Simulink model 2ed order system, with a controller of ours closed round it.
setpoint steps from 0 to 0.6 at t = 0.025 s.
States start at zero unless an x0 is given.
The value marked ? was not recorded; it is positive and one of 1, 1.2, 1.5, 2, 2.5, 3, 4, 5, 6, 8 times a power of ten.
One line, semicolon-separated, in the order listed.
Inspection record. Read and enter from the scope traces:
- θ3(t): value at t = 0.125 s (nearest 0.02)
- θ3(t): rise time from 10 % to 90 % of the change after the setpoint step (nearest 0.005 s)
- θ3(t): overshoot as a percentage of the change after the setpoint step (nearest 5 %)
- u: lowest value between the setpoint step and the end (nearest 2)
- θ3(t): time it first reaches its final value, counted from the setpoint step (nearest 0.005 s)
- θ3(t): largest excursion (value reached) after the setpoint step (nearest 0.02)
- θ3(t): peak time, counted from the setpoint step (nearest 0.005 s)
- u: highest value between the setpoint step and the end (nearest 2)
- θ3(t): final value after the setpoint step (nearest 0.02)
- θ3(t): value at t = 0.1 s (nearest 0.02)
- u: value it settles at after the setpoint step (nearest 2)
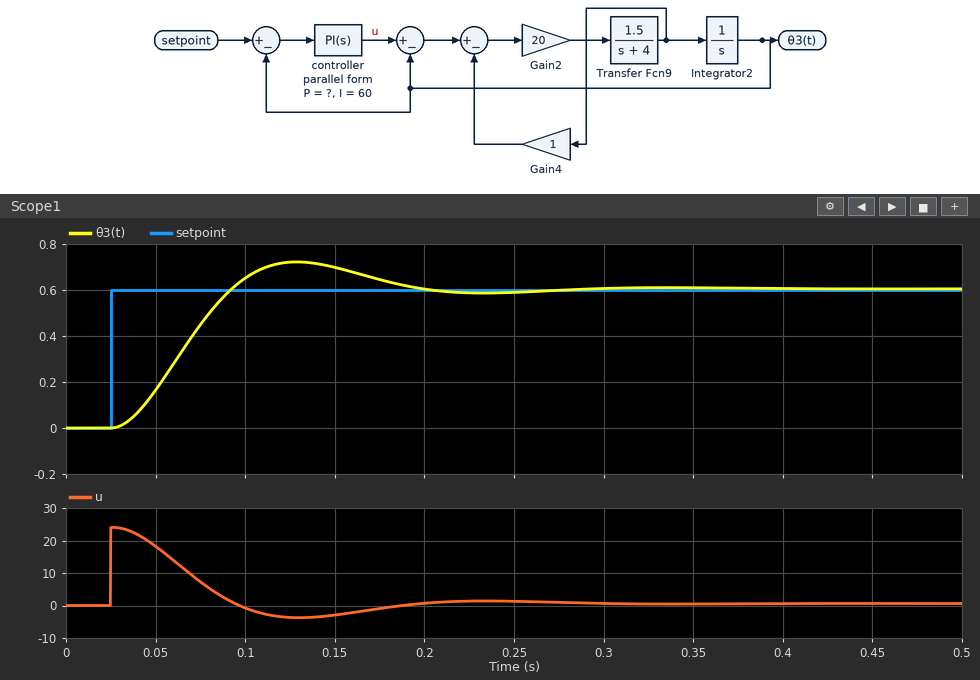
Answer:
0.72; 0.045 s; 20 %; -4; 0.065 s; 0.72; 0.105 s; 24; 0.60; 0.66; 0
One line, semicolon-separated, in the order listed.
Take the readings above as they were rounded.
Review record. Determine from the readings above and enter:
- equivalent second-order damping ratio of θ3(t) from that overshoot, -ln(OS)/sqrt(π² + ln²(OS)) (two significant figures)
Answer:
0.46
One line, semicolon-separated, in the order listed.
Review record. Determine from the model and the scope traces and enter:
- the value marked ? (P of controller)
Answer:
40
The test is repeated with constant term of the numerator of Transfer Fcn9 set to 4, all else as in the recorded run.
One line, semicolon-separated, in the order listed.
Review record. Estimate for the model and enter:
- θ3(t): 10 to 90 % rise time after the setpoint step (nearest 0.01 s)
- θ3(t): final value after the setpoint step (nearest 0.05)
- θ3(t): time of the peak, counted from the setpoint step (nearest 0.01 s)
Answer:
0.04 s; 0.60; 0.08 s
